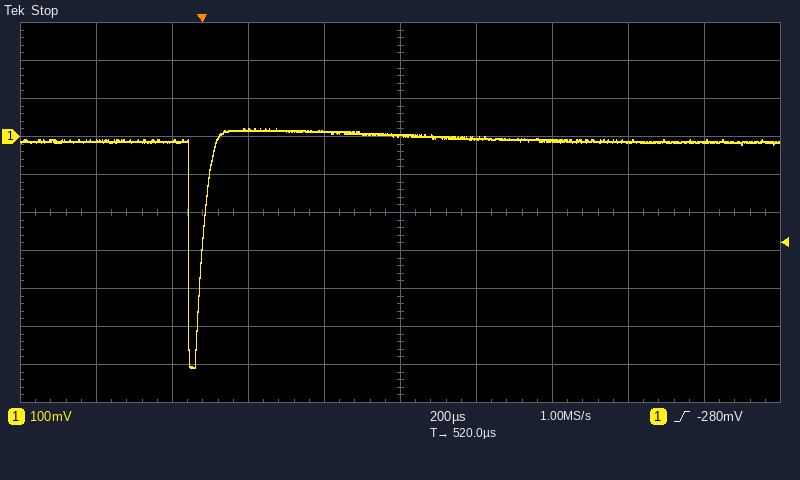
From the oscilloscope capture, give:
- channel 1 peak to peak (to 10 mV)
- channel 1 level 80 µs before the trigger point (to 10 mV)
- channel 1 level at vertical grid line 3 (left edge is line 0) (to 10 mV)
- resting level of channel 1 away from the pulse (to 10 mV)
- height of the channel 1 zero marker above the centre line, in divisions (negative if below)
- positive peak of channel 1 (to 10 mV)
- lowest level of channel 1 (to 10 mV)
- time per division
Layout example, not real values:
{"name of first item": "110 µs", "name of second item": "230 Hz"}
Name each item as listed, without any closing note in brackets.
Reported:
{"channel 1 peak to peak": "630 mV", "channel 1 level 80 µs before the trigger point": "-10 mV", "channel 1 level at vertical grid line 3 (left edge is line 0)": "20 mV", "resting level of channel 1 away from the pulse": "-10 mV", "height of the channel 1 zero marker above the centre line, in divisions": "+2.0 div", "positive peak of channel 1": "20 mV", "lowest level of channel 1": "-610 mV", "time per division": "200 µs"}
